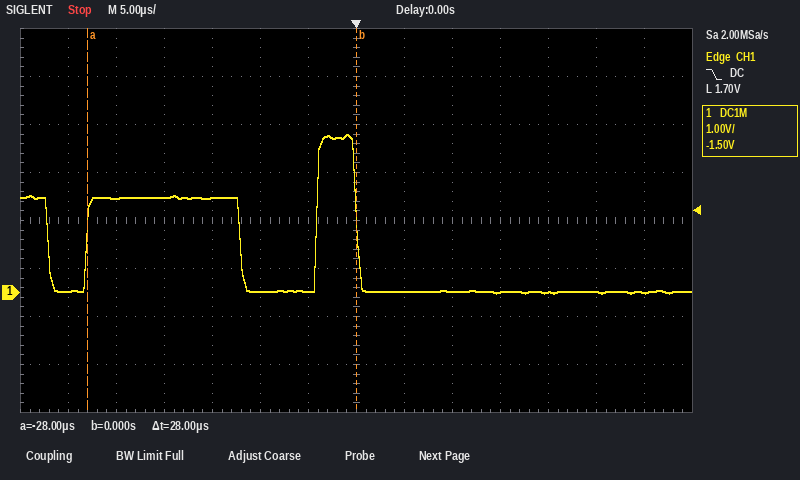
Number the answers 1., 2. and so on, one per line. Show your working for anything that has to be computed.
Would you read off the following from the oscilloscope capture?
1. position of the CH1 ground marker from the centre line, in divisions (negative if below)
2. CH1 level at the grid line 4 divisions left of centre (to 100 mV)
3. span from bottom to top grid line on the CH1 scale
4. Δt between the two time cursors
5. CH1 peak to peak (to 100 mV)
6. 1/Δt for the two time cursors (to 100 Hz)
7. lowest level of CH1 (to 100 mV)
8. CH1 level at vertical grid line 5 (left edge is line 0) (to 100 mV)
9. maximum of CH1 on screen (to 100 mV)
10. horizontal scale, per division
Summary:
1. -1.5 div
2. 2.0 V
3. 8 V
4. 28 µs
5. 3.3 V − (0.0 V) = 3.3 V
6. 1 / 28 µs ≈ 35.7 kHz
7. 0.0 V
8. 0.0 V
9. 3.3 V
10. 5 µs
